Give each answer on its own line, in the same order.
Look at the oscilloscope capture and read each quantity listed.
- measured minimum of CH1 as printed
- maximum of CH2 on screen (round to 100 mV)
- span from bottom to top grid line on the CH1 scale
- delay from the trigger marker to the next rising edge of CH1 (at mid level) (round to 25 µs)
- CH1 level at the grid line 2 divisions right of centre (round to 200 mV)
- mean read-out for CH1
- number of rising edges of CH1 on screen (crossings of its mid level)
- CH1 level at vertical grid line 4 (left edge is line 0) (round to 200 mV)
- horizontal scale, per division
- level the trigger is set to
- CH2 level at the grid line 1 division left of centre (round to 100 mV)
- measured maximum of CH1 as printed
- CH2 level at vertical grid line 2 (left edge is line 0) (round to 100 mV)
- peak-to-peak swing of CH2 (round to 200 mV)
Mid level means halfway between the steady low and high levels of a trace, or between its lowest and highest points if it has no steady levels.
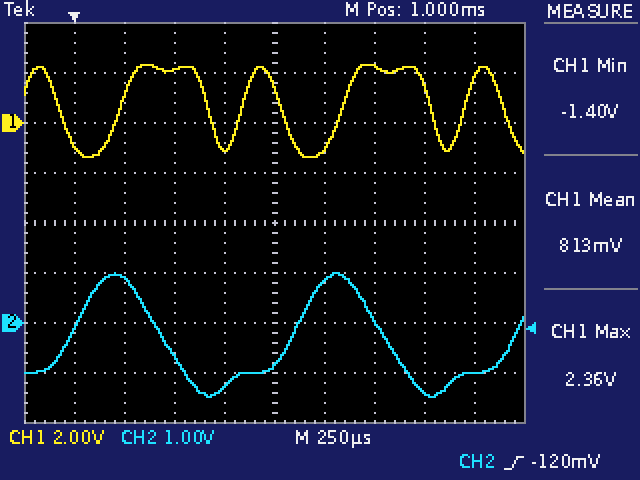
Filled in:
-1.40 V
1.0 V
16 V
225 µs
2.2 V
813 mV
4
-1.0 V
250 µs
-120 mV
-1.3 V
2.36 V
900 mV
2.4 V
